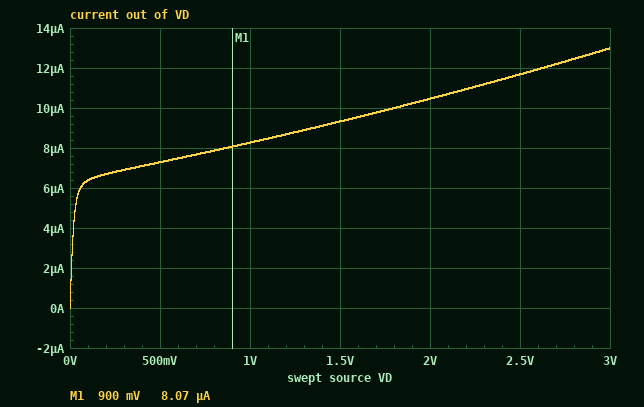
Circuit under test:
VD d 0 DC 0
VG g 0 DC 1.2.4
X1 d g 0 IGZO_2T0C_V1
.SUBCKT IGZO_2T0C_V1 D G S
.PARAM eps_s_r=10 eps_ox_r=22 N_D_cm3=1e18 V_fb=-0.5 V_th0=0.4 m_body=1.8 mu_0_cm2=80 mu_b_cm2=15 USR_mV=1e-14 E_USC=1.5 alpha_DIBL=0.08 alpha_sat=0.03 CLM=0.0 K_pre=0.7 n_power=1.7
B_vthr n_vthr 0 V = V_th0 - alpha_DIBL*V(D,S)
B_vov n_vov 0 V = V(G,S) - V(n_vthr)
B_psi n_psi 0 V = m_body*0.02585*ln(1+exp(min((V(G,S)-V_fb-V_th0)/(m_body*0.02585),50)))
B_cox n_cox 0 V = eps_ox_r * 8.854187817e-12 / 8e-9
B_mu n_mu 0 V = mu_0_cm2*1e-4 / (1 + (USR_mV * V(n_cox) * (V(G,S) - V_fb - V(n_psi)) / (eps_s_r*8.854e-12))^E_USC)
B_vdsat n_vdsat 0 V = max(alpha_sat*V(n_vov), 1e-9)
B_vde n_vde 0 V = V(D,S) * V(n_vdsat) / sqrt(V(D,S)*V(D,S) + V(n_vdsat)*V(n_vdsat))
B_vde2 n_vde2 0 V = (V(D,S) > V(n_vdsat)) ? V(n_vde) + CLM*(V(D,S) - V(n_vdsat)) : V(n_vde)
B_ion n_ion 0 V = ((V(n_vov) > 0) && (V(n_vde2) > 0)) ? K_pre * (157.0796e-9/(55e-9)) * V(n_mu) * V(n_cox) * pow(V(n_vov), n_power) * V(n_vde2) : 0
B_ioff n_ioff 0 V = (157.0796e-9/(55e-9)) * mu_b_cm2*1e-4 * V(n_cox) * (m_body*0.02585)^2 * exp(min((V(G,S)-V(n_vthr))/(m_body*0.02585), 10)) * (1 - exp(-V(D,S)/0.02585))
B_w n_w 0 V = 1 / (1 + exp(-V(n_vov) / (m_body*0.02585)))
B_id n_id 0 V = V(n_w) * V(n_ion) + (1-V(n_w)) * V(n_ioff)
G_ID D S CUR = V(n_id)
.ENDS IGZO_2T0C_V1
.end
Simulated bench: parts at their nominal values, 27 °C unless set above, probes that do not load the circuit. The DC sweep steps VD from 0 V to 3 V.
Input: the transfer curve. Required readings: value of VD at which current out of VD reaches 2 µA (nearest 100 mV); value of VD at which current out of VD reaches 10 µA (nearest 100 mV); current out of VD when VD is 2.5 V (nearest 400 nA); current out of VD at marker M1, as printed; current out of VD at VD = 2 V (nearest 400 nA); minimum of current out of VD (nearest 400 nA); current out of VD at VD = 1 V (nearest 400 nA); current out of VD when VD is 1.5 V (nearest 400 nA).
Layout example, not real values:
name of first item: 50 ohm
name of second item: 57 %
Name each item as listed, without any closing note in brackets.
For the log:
value of VD at which current out of VD reaches 2 µA: 0 V
value of VD at which current out of VD reaches 10 µA: 1.8 V
current out of VD when VD is 2.5 V: 11.6 µA
current out of VD at marker M1, as printed: 8.07 µA
current out of VD at VD = 2 V: 10.4 µA
minimum of current out of VD: 0 A
current out of VD at VD = 1 V: 8.4 µA
current out of VD when VD is 1.5 V: 9.2 µA
